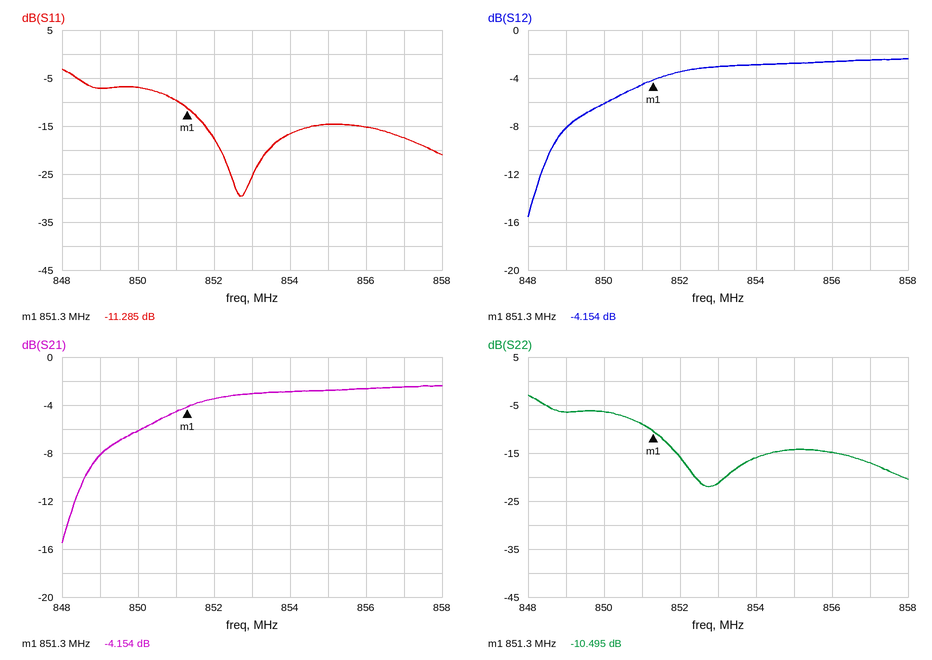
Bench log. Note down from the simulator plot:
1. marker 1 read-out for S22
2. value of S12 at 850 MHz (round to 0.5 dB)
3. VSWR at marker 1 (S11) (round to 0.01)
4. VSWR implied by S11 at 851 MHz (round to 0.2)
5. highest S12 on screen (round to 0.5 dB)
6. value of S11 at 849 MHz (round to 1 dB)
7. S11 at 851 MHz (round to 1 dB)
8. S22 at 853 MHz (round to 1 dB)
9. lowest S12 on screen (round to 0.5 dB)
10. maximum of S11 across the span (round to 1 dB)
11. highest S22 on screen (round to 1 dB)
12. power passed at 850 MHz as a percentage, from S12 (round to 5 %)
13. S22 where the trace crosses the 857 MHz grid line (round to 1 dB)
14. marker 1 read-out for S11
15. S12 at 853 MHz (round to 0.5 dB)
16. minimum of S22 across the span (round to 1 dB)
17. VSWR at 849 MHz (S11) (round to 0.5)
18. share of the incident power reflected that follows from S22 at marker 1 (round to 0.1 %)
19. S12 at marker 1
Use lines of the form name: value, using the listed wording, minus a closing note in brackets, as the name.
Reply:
marker 1 read-out for S22: -10.495 dB
value of S12 at 850 MHz: -6.0 dB
VSWR at marker 1 (S11): 1.75
VSWR implied by S11 at 851 MHz: 2.0
highest S12 on screen: -2.5 dB
value of S11 at 849 MHz: -7 dB
S11 at 851 MHz: -10 dB
S22 at 853 MHz: -21 dB
lowest S12 on screen: -15.5 dB
maximum of S11 across the span: -3 dB
highest S22 on screen: -3 dB
power passed at 850 MHz as a percentage, from S12: 25 %
S22 where the trace crosses the 857 MHz grid line: -17 dB
marker 1 read-out for S11: -11.285 dB
S12 at 853 MHz: -3.0 dB
minimum of S22 across the span: -22 dB
VSWR at 849 MHz (S11): 2.5
share of the incident power reflected that follows from S22 at marker 1: 8.9 %
S12 at marker 1: -4.154 dB
